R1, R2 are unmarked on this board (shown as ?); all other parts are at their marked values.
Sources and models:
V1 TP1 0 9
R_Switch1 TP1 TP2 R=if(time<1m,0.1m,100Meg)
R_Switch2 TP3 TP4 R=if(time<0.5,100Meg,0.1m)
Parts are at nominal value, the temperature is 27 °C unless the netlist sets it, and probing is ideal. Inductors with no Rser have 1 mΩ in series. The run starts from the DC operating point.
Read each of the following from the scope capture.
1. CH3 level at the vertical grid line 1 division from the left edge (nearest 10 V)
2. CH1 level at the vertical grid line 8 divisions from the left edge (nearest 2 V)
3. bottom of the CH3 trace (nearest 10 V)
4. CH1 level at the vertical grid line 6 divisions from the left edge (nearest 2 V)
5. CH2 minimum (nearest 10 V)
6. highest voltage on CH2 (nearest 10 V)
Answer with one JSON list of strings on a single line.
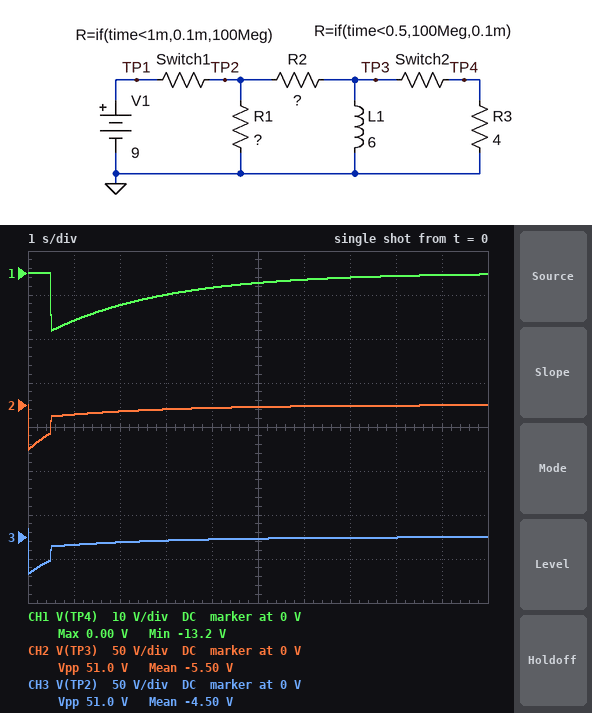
["-10 V", "0 V", "-40 V", "-2 V", "-50 V", "0 V"]
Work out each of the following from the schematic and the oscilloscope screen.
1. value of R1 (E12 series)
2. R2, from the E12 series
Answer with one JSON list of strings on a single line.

["4.7 Ω", "1 Ω"]
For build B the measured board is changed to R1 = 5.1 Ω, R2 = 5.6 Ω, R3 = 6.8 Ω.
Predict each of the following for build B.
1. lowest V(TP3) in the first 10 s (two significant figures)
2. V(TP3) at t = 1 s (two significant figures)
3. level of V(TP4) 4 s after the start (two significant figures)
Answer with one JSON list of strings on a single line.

["-17 V", "-1.9 V", "-240 mV"]
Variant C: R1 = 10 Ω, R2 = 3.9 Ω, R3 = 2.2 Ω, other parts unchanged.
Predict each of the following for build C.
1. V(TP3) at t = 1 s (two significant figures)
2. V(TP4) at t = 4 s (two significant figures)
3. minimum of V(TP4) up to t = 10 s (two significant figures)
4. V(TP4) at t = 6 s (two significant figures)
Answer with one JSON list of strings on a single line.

["-1.2 V", "-460 mV", "-1.4 V", "-240 mV"]
